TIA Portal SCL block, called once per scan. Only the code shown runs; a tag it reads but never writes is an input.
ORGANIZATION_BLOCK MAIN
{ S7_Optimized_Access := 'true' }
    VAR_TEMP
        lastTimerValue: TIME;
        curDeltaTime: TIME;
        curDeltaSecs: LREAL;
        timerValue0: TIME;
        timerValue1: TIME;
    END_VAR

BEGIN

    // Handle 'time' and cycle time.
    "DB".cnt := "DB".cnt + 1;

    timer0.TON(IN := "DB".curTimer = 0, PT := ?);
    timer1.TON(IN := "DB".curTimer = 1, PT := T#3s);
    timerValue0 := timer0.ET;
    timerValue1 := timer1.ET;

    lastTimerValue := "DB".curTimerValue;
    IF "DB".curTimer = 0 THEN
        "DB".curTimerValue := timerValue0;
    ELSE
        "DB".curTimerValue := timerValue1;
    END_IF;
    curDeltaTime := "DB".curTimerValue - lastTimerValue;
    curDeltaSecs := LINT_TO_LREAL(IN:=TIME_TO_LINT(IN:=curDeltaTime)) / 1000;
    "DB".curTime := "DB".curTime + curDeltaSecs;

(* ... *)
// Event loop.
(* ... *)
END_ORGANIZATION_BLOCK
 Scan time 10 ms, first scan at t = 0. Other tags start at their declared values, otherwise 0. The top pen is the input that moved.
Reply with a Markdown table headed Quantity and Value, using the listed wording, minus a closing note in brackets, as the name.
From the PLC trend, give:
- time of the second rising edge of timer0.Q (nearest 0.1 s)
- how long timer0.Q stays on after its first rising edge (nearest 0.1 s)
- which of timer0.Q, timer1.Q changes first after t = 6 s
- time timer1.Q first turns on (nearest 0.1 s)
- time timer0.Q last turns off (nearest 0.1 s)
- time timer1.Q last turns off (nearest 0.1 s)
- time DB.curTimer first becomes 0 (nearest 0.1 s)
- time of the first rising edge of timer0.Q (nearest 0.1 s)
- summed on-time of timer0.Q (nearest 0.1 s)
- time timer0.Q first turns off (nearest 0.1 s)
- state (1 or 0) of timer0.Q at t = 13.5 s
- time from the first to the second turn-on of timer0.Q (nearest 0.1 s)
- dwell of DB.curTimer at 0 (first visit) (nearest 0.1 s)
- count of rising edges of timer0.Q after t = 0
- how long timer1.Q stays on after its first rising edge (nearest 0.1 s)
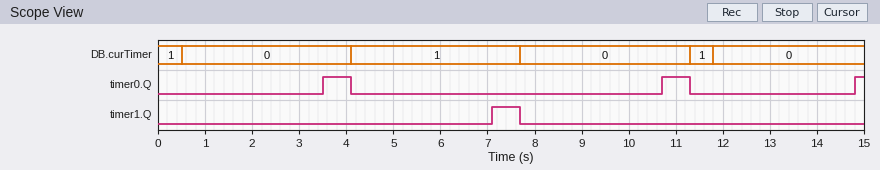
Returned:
| Quantity | Value |
|---|---|
| time of the second rising edge of timer0.Q | 10.7 s |
| how long timer0.Q stays on after its first rising edge | 0.6 s |
| which of timer0.Q, timer1.Q changes first after t = 6 s | timer1.Q |
| time timer1.Q first turns on | 7.1 s |
| time timer0.Q last turns off | 11.3 s |
| time timer1.Q last turns off | 7.7 s |
| time DB.curTimer first becomes 0 | 0.5 s |
| time of the first rising edge of timer0.Q | 3.5 s |
| summed on-time of timer0.Q | 1.4 s |
| time timer0.Q first turns off | 4.1 s |
| state (1 or 0) of timer0.Q at t = 13.5 s | 0 |
| time from the first to the second turn-on of timer0.Q | 7.2 s |
| dwell of DB.curTimer at 0 (first visit) | 3.6 s |
| count of rising edges of timer0.Q after t = 0 | 3 |
| how long timer1.Q stays on after its first rising edge | 0.6 s |
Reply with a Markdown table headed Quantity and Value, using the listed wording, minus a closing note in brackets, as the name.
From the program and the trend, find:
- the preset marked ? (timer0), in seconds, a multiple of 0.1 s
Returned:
| Quantity | Value |
|---|---|
| the preset marked ? (timer0), in seconds, a multiple of 0.1 s | 3.0 s |
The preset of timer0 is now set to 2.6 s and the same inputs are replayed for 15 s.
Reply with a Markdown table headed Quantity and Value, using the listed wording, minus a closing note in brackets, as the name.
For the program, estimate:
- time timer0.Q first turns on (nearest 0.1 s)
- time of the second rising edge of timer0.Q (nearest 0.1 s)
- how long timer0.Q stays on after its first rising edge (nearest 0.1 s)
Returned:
| Quantity | Value |
|---|---|
| time timer0.Q first turns on | 3.1 s |
| time of the second rising edge of timer0.Q | 10.3 s |
| how long timer0.Q stays on after its first rising edge | 1.0 s |
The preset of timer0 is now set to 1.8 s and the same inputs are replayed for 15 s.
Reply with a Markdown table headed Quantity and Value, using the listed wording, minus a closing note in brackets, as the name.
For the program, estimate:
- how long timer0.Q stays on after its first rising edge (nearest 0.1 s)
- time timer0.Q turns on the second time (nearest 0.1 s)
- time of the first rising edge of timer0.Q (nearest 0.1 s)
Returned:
| Quantity | Value |
|---|---|
| how long timer0.Q stays on after its first rising edge | 1.8 s |
| time timer0.Q turns on the second time | 9.5 s |
| time of the first rising edge of timer0.Q | 2.3 s |
